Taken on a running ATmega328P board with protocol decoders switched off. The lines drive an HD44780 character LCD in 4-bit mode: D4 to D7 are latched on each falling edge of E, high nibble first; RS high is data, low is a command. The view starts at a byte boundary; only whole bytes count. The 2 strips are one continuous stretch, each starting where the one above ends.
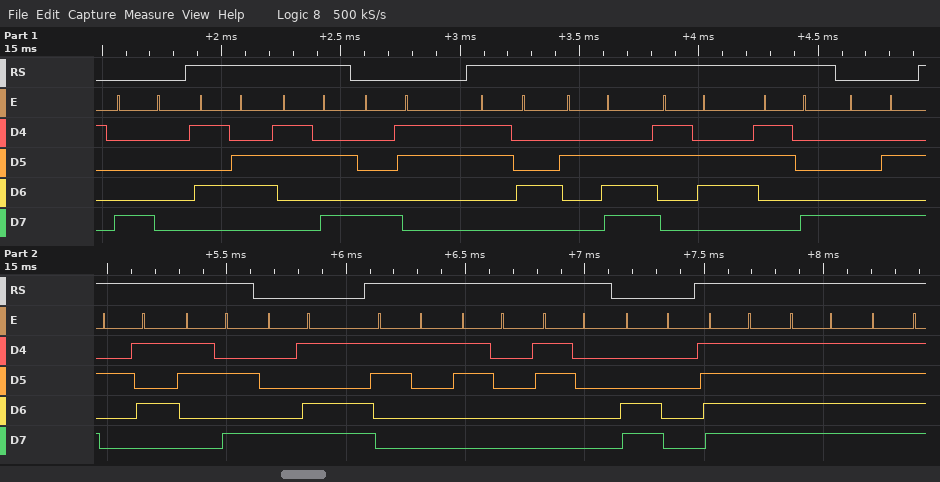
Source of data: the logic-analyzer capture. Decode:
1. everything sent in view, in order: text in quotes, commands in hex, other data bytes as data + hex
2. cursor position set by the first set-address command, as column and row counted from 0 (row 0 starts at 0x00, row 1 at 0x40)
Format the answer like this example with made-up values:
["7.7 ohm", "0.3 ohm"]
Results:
["0x80 \"V:\" 0x83 \"4.68\" 0x8A \"%:\" 0x8D \"100\" 0xC0 data FF FF FF", "column 0, row 0"]
